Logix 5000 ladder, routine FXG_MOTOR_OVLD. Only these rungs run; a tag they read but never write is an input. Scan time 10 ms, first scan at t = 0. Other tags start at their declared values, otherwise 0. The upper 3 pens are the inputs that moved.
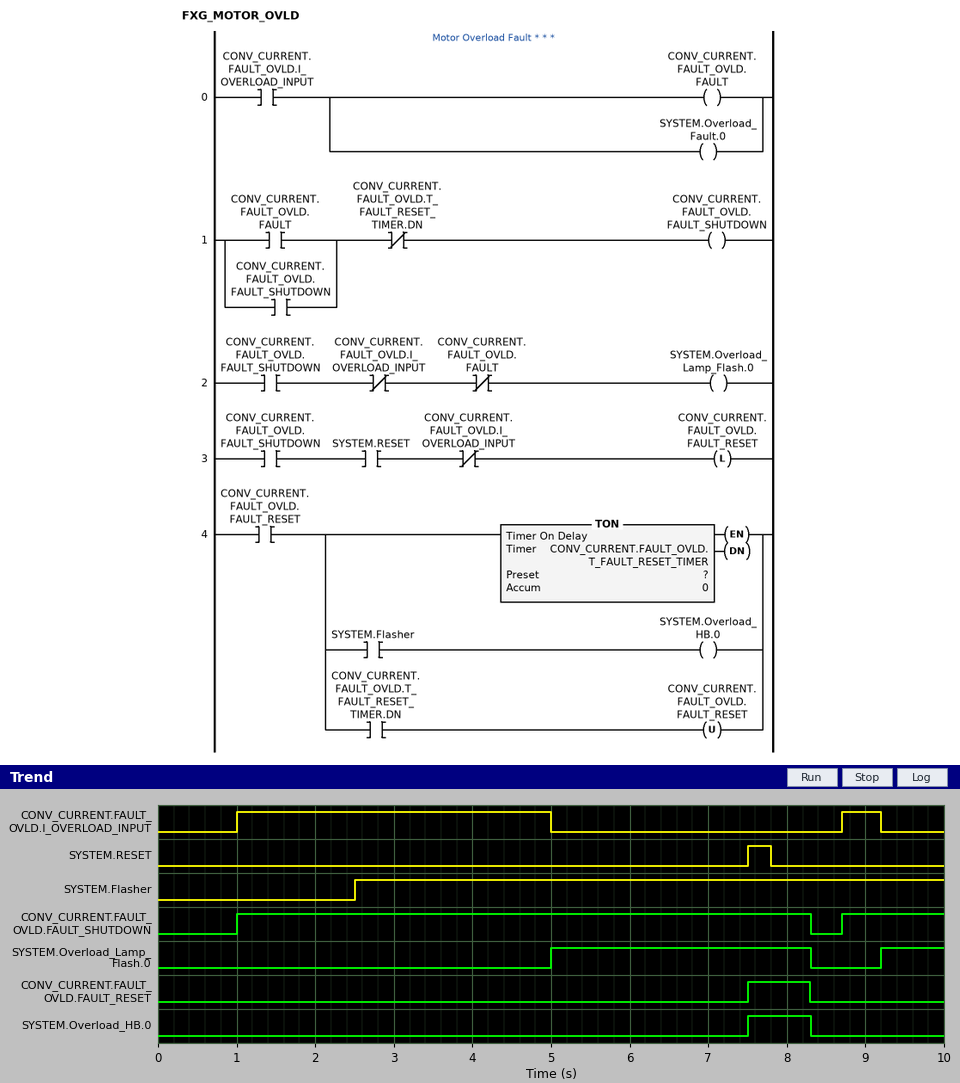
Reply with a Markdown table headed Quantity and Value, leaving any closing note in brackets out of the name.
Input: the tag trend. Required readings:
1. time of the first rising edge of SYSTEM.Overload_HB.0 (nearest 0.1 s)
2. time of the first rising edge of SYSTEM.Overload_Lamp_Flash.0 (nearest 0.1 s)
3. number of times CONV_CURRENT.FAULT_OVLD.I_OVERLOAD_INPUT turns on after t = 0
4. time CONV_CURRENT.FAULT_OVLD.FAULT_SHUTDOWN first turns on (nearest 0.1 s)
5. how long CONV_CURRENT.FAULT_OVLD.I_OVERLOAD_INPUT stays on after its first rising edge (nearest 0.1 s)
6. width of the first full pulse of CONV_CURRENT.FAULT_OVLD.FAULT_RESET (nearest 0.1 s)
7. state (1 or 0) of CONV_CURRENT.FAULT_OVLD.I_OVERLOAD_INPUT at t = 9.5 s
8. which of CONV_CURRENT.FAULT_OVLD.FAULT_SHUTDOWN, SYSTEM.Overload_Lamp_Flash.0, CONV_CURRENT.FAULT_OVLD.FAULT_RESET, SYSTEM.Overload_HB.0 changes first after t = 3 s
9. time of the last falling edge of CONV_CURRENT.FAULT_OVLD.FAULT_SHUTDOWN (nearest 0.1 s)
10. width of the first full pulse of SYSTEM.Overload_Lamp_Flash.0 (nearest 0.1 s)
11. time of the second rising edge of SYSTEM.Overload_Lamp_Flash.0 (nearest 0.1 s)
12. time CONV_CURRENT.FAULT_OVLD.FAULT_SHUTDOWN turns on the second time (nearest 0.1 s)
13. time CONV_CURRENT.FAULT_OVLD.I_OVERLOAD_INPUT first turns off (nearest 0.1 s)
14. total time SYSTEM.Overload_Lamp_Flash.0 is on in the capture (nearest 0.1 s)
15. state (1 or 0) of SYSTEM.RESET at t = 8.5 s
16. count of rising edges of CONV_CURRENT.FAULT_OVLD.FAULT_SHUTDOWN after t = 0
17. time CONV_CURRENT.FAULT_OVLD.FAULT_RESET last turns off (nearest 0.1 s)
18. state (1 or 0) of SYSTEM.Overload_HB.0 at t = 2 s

| Quantity | Value |
|---|---|
| time of the first rising edge of SYSTEM.Overload_HB.0 | 7.5 s |
| time of the first rising edge of SYSTEM.Overload_Lamp_Flash.0 | 5.0 s |
| number of times CONV_CURRENT.FAULT_OVLD.I_OVERLOAD_INPUT turns on after t = 0 | 2 |
| time CONV_CURRENT.FAULT_OVLD.FAULT_SHUTDOWN first turns on | 1.0 s |
| how long CONV_CURRENT.FAULT_OVLD.I_OVERLOAD_INPUT stays on after its first rising edge | 4.0 s |
| width of the first full pulse of CONV_CURRENT.FAULT_OVLD.FAULT_RESET | 0.8 s |
| state (1 or 0) of CONV_CURRENT.FAULT_OVLD.I_OVERLOAD_INPUT at t = 9.5 s | 0 |
| which of CONV_CURRENT.FAULT_OVLD.FAULT_SHUTDOWN, SYSTEM.Overload_Lamp_Flash.0, CONV_CURRENT.FAULT_OVLD.FAULT_RESET, SYSTEM.Overload_HB.0 changes first after t = 3 s | SYSTEM.Overload_Lamp_Flash.0 |
| time of the last falling edge of CONV_CURRENT.FAULT_OVLD.FAULT_SHUTDOWN | 8.3 s |
| width of the first full pulse of SYSTEM.Overload_Lamp_Flash.0 | 3.3 s |
| time of the second rising edge of SYSTEM.Overload_Lamp_Flash.0 | 9.2 s |
| time CONV_CURRENT.FAULT_OVLD.FAULT_SHUTDOWN turns on the second time | 8.7 s |
| time CONV_CURRENT.FAULT_OVLD.I_OVERLOAD_INPUT first turns off | 5.0 s |
| total time SYSTEM.Overload_Lamp_Flash.0 is on in the capture | 4.1 s |
| state (1 or 0) of SYSTEM.RESET at t = 8.5 s | 0 |
| count of rising edges of CONV_CURRENT.FAULT_OVLD.FAULT_SHUTDOWN after t = 0 | 2 |
| time CONV_CURRENT.FAULT_OVLD.FAULT_RESET last turns off | 8.3 s |
| state (1 or 0) of SYSTEM.Overload_HB.0 at t = 2 s | 0 |
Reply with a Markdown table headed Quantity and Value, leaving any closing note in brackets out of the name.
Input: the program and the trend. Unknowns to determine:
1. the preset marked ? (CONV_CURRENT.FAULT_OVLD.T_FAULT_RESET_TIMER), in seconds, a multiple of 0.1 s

| Quantity | Value |
|---|---|
| the preset marked ? (CONV_CURRENT.FAULT_OVLD.T_FAULT_RESET_TIMER), in seconds, a multiple of 0.1 s | 0.8 s |
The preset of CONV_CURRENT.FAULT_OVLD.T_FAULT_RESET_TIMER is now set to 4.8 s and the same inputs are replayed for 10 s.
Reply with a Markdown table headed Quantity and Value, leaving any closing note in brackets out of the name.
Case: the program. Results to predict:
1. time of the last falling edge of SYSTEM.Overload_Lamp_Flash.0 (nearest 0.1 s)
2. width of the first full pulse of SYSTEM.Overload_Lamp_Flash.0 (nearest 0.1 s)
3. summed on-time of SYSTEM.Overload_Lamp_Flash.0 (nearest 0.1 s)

| Quantity | Value |
|---|---|
| time of the last falling edge of SYSTEM.Overload_Lamp_Flash.0 | 8.7 s |
| width of the first full pulse of SYSTEM.Overload_Lamp_Flash.0 | 3.7 s |
| summed on-time of SYSTEM.Overload_Lamp_Flash.0 | 4.5 s |
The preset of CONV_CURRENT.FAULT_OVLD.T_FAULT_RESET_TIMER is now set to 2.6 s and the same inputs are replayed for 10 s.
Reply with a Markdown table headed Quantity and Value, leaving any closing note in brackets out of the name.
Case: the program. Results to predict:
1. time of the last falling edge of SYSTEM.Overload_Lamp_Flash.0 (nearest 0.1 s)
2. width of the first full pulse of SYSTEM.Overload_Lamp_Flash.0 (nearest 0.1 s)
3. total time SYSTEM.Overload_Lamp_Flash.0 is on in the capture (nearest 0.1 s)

| Quantity | Value |
|---|---|
| time of the last falling edge of SYSTEM.Overload_Lamp_Flash.0 | 8.7 s |
| width of the first full pulse of SYSTEM.Overload_Lamp_Flash.0 | 3.7 s |
| total time SYSTEM.Overload_Lamp_Flash.0 is on in the capture | 4.5 s |
